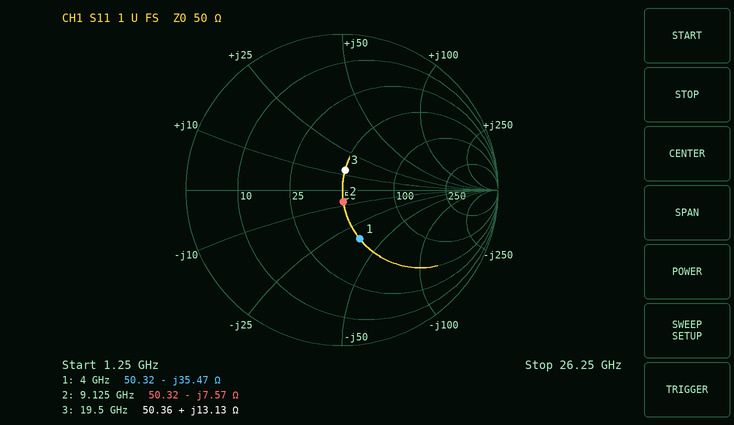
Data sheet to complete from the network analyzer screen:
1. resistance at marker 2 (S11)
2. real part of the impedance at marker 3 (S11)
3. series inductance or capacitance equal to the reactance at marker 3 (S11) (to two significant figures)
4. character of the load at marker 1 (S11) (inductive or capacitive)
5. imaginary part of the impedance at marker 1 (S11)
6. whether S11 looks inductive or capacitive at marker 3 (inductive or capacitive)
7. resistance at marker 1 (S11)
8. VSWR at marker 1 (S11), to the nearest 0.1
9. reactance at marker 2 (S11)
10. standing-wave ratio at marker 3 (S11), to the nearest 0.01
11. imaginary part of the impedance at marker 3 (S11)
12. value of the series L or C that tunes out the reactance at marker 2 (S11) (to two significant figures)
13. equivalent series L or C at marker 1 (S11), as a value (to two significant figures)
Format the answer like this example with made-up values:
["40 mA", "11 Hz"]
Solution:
["50.32 Ω", "50.36 Ω", "110 pH", "capacitive", "-35.47 Ω", "inductive", "50.32 Ω", "2.0", "-7.57 Ω", "1.30", "+13.13 Ω", "130 pH", "1.1 pF"]
